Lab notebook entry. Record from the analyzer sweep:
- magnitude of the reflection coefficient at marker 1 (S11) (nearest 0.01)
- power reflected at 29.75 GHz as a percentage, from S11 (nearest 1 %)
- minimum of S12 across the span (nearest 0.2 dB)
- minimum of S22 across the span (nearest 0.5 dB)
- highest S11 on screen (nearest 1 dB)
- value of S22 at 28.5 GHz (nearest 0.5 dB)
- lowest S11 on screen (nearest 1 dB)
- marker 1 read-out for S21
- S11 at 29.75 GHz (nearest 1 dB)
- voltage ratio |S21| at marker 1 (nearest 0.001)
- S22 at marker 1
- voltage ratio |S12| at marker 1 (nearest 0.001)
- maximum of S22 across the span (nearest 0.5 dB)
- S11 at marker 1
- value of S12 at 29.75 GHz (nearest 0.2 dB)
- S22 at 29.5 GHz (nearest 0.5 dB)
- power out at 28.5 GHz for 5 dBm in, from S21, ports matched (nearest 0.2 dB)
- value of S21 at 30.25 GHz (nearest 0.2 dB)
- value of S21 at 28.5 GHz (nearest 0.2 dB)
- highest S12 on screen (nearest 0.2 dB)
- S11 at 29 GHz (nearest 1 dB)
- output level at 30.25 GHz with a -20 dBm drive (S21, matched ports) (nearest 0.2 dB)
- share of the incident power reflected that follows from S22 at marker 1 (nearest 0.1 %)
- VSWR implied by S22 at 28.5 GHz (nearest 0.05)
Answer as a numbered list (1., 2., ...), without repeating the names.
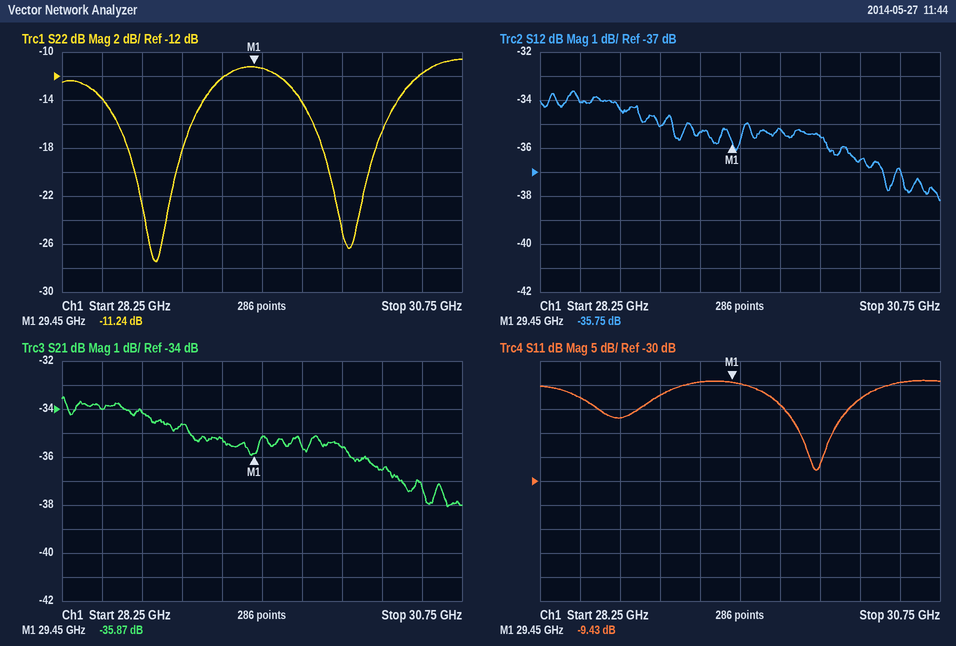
1. 0.34
2. 4 %
3. -38.2 dB
4. -27.5 dB
5. -9 dB
6. -14.0 dB
7. -28 dB
8. -35.87 dB
9. -14 dB
10. 0.016
11. -11.24 dB
12. 0.016
13. -10.5 dB
14. -9.43 dB
15. -35.2 dB
16. -11.5 dB
17. -29.0 dBm
18. -36.6 dB
19. -34.0 dB
20. -33.6 dB
21. -12 dB
22. -56.6 dBm
23. 7.5 %
24. 1.50
